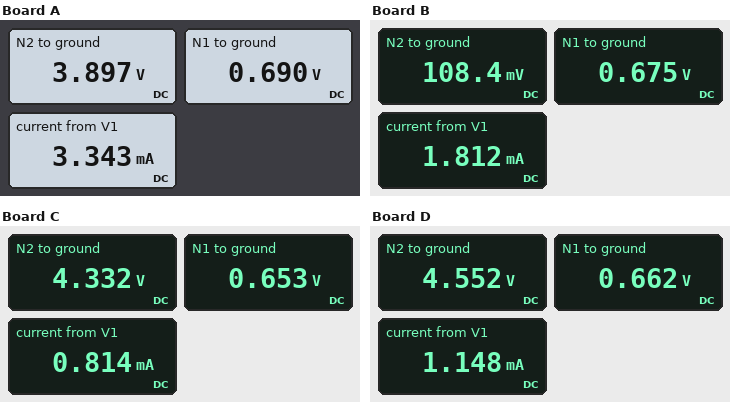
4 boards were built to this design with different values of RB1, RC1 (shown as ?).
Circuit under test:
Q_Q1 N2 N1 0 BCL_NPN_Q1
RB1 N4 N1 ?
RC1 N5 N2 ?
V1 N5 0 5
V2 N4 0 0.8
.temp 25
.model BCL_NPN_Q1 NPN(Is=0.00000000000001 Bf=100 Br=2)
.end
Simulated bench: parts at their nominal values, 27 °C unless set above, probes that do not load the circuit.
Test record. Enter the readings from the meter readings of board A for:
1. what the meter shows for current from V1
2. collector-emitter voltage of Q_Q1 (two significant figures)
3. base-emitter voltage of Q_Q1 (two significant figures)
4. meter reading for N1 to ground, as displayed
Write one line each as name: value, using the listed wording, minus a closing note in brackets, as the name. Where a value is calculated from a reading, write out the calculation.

what the meter shows for current from V1: 3.343 mA
collector-emitter voltage of Q_Q1: 3.897 V = 3.9 V
base-emitter voltage of Q_Q1: 690 mV = 690 mV
meter reading for N1 to ground, as displayed: 0.690 V
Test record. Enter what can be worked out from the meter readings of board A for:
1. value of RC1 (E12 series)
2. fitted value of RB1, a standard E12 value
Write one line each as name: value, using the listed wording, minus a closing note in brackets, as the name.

value of RC1: 330 Ω
fitted value of RB1, a standard E12 value: 3.3 kΩ
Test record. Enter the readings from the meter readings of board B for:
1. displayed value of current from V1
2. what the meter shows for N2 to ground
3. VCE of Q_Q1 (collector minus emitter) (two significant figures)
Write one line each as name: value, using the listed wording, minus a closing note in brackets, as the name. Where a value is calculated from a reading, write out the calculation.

displayed value of current from V1: 1.812 mA
what the meter shows for N2 to ground: 108.4 mV
VCE of Q_Q1 (collector minus emitter): 108.4 mV = 110 mV
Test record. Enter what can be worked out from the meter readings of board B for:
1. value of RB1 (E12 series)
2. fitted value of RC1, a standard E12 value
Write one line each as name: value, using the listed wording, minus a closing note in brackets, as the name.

value of RB1: 3.9 kΩ
fitted value of RC1, a standard E12 value: 2.7 kΩ
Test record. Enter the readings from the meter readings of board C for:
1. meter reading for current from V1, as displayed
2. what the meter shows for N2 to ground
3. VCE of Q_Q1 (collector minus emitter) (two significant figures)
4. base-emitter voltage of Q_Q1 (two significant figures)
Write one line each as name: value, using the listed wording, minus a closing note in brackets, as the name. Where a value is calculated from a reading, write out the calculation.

meter reading for current from V1, as displayed: 0.814 mA
what the meter shows for N2 to ground: 4.332 V
VCE of Q_Q1 (collector minus emitter): 4.332 V = 4.3 V
base-emitter voltage of Q_Q1: 653 mV = 650 mV
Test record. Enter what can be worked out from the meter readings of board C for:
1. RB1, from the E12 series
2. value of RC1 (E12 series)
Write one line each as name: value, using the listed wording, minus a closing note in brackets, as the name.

RB1, from the E12 series: 18 kΩ
value of RC1: 820 Ω
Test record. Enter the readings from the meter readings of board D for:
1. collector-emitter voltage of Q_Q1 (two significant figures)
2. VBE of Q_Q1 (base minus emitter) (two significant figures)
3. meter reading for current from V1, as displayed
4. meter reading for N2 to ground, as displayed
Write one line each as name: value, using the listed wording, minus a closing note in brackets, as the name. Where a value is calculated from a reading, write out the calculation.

collector-emitter voltage of Q_Q1: 4.552 V = 4.6 V
VBE of Q_Q1 (base minus emitter): 662 mV = 660 mV
meter reading for current from V1, as displayed: 1.148 mA
meter reading for N2 to ground, as displayed: 4.552 V
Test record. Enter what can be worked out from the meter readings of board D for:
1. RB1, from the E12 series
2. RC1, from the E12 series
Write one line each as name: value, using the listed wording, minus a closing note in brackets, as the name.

RB1, from the E12 series: 12 kΩ
RC1, from the E12 series: 390 Ω
